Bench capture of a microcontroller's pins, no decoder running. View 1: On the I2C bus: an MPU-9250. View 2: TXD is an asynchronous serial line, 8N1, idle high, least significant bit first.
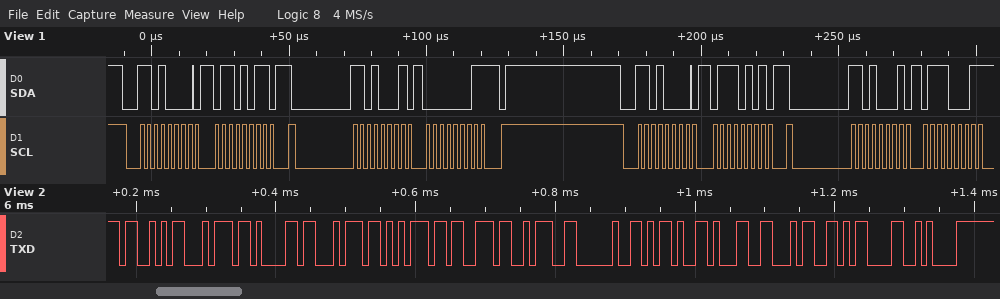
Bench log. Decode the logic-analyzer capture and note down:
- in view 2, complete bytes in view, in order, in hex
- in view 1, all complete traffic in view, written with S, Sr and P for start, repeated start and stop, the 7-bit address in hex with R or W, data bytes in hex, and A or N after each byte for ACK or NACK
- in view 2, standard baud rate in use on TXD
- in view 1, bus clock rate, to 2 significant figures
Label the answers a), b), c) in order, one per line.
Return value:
a) 0x53 0x74 0x61 0x74 0x75 0x73 0x3A 0x20 0x2D 0x31 0x34 0x0D 0x0A
b) S 68W A 6B A Sr 68R A 01 N P S 68W A 75 A Sr 68R A 71 N
c) 115200 baud
d) 400 kHz
